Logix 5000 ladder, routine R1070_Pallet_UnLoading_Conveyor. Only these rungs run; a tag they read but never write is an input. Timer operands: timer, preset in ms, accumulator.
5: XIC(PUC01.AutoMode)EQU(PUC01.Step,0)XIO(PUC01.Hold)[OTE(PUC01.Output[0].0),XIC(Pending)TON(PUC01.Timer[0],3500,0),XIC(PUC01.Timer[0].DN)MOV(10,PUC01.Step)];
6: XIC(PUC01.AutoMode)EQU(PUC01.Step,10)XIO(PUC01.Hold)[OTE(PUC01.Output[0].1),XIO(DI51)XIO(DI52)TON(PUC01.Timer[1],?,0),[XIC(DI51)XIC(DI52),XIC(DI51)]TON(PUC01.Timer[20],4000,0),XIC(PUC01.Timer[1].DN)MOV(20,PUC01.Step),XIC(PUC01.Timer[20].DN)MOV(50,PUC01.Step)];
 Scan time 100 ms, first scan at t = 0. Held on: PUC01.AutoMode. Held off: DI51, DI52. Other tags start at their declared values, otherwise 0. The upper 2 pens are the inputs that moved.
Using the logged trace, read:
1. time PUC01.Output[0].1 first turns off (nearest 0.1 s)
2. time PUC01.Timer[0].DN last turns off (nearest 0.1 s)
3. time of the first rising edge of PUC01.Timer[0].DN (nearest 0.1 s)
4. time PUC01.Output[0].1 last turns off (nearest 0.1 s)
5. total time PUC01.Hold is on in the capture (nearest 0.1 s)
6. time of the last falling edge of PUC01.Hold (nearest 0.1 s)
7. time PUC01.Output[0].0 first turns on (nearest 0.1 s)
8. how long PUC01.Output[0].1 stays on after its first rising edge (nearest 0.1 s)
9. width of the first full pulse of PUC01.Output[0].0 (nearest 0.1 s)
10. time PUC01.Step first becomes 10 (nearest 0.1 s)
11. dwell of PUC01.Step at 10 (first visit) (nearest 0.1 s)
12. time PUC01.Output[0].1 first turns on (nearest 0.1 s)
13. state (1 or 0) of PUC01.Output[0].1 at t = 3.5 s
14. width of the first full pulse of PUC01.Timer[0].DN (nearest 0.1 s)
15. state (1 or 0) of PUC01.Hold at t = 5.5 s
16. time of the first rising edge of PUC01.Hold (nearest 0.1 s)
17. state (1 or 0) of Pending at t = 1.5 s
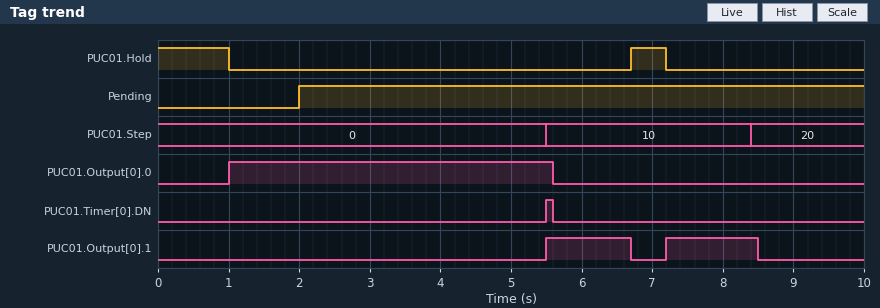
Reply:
6.7 s
5.6 s
5.5 s
8.5 s
1.5 s
7.2 s
1.0 s
1.2 s
4.6 s
5.5 s
2.9 s
5.5 s
0
0.1 s
0
6.7 s
0
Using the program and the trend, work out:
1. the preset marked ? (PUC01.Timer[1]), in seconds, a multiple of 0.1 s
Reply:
1.2 s
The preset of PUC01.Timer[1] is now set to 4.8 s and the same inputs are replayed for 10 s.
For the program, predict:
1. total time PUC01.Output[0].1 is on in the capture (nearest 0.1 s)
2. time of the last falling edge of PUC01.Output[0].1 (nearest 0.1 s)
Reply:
4.0 s
6.7 s
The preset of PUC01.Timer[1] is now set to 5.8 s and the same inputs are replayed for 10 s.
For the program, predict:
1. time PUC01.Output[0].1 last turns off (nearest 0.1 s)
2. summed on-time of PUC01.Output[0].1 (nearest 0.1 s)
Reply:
6.7 s
4.0 s
